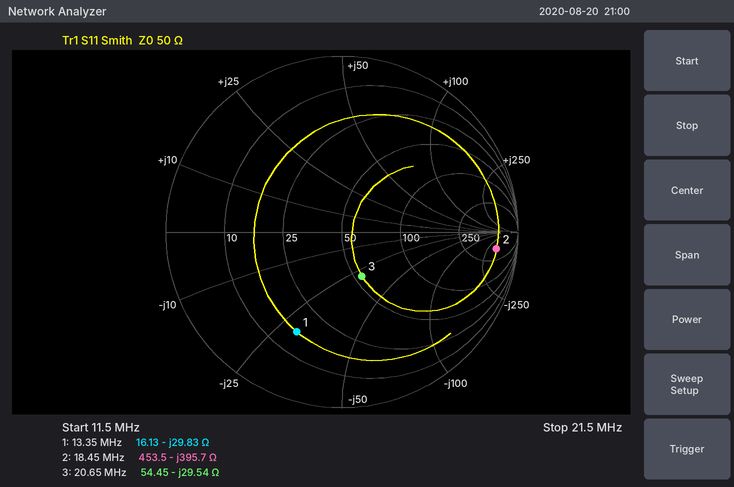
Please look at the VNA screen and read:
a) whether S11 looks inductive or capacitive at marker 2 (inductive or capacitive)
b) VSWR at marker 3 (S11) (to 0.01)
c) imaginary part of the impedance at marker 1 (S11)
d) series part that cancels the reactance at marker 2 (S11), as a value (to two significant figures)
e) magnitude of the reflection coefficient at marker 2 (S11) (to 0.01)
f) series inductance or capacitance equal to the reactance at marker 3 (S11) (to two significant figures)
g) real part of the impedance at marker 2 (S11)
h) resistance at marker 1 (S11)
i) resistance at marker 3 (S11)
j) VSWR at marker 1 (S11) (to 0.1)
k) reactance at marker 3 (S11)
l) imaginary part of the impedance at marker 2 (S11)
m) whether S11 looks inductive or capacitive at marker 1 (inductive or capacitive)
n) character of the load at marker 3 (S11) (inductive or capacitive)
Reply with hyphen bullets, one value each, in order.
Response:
- capacitive
- 1.76
- -29.83 Ω
- 3.4 µH
- 0.88
- 260 pF
- 453.5 Ω
- 16.13 Ω
- 54.45 Ω
- 4.3
- -29.54 Ω
- -395.7 Ω
- capacitive
- capacitive
